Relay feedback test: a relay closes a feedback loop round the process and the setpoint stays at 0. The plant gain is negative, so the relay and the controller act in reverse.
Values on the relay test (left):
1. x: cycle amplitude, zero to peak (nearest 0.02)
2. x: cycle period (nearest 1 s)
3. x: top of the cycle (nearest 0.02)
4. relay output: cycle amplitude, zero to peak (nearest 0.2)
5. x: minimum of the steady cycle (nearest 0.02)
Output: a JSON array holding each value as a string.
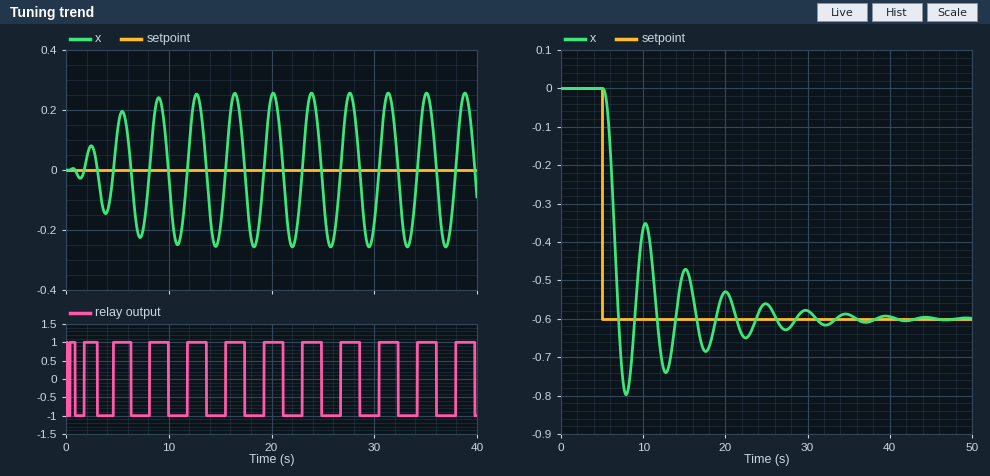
["0.26", "4 s", "0.26", "1.0", "-0.26"]
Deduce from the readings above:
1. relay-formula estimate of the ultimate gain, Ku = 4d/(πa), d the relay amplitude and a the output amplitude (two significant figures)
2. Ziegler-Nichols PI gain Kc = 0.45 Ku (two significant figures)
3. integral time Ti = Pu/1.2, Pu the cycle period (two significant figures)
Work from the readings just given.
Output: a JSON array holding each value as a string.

["4.9", "2.2", "3.3 s"]
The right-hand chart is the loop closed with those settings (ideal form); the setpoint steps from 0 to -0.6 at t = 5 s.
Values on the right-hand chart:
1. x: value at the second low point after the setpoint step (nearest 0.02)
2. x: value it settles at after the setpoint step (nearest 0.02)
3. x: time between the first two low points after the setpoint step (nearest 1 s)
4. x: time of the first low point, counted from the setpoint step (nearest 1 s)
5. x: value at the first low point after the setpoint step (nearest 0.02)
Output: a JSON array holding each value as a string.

["-0.74", "-0.60", "5 s", "3 s", "-0.80"]
